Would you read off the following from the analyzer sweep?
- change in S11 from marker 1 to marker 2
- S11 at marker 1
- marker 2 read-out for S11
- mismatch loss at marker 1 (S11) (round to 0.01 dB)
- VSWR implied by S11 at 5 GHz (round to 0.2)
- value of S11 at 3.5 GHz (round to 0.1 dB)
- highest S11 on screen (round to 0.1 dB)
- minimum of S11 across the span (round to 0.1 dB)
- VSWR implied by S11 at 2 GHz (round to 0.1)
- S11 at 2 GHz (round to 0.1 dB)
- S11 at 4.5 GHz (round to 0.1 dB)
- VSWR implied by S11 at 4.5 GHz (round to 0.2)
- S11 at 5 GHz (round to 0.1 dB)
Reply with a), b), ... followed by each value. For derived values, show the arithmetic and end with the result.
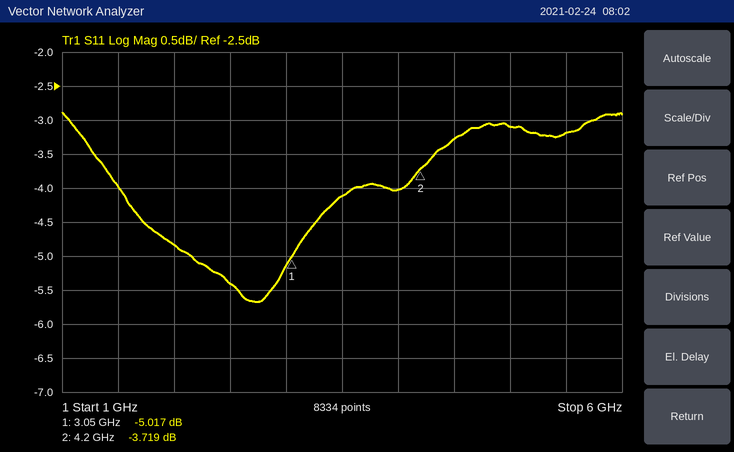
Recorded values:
a) -3.719 − (-5.017) = 1.298 dB
b) -5.017 dB
c) -3.719 dB
d) −10 log10(1 − 10^(-5.017/10)) ≈ 1.64 dB
e) |Γ| = 10^(-3.1/20) = 0.6998; VSWR = (1 + 0.6998)/(1 − 0.6998) ≈ 5.66, so 5.6 to the nearest 0.2
f) -4.1 dB
g) -2.9 dB
h) -5.7 dB
i) |Γ| = 10^(-4.8/20) = 0.5754; VSWR = (1 + 0.5754)/(1 − 0.5754) ≈ 3.7
j) -4.8 dB
k) -3.3 dB
l) |Γ| = 10^(-3.3/20) = 0.6839; VSWR = (1 + 0.6839)/(1 − 0.6839) ≈ 5.33, so 5.4 to the nearest 0.2
m) -3.1 dB
